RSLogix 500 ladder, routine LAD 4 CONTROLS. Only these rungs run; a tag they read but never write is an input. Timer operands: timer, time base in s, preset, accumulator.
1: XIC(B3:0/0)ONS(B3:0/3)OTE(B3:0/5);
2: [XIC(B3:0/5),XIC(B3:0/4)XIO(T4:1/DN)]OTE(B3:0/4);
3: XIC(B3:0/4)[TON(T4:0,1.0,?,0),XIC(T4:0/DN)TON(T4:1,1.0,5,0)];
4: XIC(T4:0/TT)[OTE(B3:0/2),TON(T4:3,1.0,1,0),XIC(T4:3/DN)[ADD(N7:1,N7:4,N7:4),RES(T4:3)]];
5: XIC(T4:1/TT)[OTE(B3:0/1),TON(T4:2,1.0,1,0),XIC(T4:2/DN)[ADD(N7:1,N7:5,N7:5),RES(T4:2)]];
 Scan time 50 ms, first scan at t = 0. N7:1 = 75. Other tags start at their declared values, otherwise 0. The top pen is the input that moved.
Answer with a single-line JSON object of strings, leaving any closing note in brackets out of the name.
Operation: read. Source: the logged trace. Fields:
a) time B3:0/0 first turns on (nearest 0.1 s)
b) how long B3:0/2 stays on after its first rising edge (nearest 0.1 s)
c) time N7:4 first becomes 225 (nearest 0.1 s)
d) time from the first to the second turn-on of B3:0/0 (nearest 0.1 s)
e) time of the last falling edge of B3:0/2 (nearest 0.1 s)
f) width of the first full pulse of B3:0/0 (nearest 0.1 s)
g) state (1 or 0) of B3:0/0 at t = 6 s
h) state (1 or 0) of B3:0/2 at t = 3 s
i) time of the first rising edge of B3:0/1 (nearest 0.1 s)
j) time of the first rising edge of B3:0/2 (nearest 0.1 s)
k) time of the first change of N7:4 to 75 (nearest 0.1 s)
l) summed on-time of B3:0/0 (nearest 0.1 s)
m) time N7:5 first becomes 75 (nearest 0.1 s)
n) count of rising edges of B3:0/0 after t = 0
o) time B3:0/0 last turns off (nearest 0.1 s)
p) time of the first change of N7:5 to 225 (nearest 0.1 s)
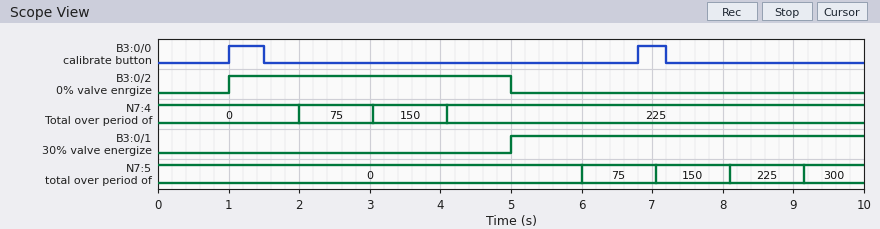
{"time B3:0/0 first turns on": "1.0 s", "how long B3:0/2 stays on after its first rising edge": "4.0 s", "time N7:4 first becomes 225": "4.1 s", "time from the first to the second turn-on of B3:0/0": "5.8 s", "time of the last falling edge of B3:0/2": "5.0 s", "width of the first full pulse of B3:0/0": "0.5 s", "state (1 or 0) of B3:0/0 at t = 6 s": "0", "state (1 or 0) of B3:0/2 at t = 3 s": "1", "time of the first rising edge of B3:0/1": "5.0 s", "time of the first rising edge of B3:0/2": "1.0 s", "time of the first change of N7:4 to 75": "2.0 s", "summed on-time of B3:0/0": "0.9 s", "time N7:5 first becomes 75": "6.0 s", "count of rising edges of B3:0/0 after t = 0": "2", "time B3:0/0 last turns off": "7.2 s", "time of the first change of N7:5 to 225": "8.1 s"}
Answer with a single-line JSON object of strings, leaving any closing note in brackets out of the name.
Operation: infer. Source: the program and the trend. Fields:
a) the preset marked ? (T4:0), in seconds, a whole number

{"the preset marked ? (T4:0), in seconds, a whole number": "4 s"}
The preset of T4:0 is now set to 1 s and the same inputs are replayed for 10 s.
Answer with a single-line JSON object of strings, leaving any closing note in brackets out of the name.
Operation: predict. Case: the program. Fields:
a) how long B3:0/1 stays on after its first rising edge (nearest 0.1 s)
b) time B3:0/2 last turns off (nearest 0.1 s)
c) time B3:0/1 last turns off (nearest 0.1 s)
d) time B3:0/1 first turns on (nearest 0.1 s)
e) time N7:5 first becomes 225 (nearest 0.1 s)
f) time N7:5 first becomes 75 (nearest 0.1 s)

{"how long B3:0/1 stays on after its first rising edge": "5.0 s", "time B3:0/2 last turns off": "2.0 s", "time B3:0/1 last turns off": "7.0 s", "time B3:0/1 first turns on": "2.0 s", "time N7:5 first becomes 225": "5.1 s", "time N7:5 first becomes 75": "3.0 s"}
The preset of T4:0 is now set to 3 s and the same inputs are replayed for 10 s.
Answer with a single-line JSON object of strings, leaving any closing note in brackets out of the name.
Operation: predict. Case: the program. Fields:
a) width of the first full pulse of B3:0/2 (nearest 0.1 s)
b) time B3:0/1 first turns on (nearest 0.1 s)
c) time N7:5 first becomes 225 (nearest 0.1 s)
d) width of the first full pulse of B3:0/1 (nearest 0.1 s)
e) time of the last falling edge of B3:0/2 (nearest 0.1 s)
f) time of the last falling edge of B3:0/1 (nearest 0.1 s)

{"width of the first full pulse of B3:0/2": "3.0 s", "time B3:0/1 first turns on": "4.0 s", "time N7:5 first becomes 225": "7.1 s", "width of the first full pulse of B3:0/1": "5.0 s", "time of the last falling edge of B3:0/2": "4.0 s", "time of the last falling edge of B3:0/1": "9.0 s"}
